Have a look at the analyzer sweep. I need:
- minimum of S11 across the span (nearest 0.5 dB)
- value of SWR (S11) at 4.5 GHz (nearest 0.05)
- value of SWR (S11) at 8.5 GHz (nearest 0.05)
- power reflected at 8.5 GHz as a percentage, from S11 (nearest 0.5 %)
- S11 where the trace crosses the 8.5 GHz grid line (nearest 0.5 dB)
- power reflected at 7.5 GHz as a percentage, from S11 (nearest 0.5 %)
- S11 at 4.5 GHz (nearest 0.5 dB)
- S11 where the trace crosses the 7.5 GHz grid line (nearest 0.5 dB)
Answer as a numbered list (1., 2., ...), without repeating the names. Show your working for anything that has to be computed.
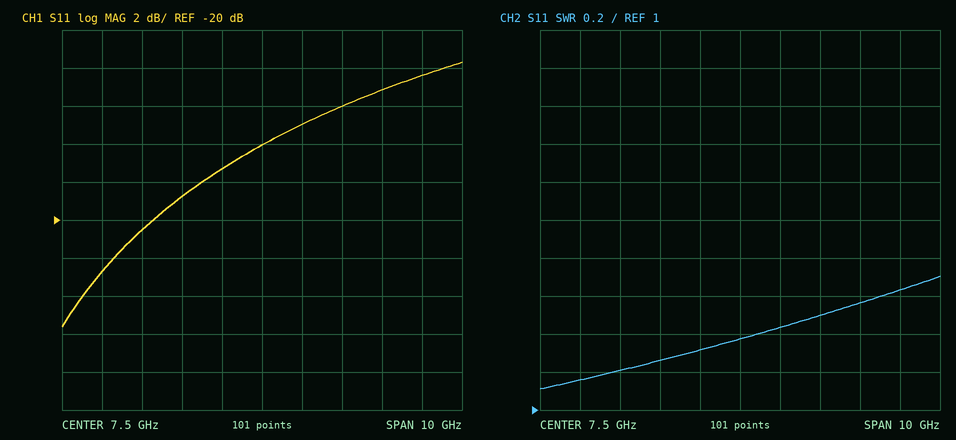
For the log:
1. -25.5 dB
2. 1.20
3. 1.45
4. 10^(-15/10) ≈ 3.16 %, so 3.0 % to the nearest 0.5 %
5. -15.0 dB
6. 10^(-16/10) ≈ 2.5 %
7. -20.5 dB
8. -16.0 dB
